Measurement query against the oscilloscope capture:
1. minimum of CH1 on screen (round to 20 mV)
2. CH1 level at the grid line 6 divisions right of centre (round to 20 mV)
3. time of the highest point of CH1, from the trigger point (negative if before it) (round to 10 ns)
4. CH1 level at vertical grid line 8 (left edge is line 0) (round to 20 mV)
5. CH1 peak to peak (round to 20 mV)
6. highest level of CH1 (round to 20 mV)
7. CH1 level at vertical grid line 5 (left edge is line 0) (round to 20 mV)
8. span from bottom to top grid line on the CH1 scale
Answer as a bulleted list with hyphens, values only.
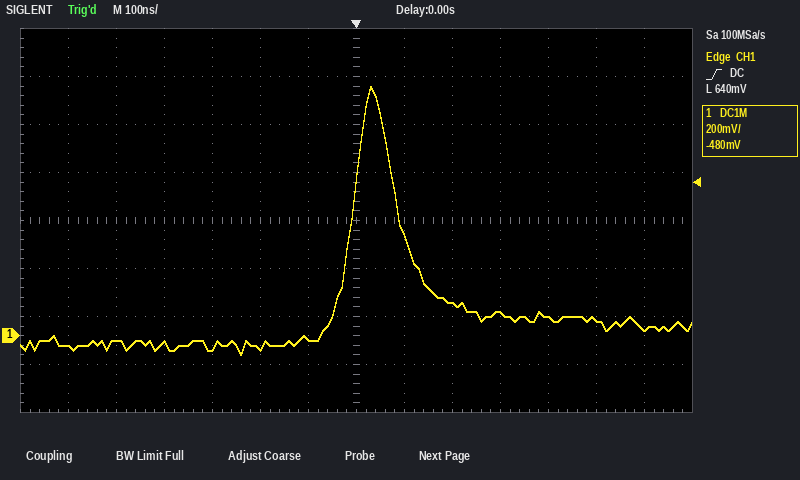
- -80 mV
- 20 mV
- +30 ns
- 420 mV
- 1.12 V
- 1.04 V
- -60 mV
- 1.6 V
